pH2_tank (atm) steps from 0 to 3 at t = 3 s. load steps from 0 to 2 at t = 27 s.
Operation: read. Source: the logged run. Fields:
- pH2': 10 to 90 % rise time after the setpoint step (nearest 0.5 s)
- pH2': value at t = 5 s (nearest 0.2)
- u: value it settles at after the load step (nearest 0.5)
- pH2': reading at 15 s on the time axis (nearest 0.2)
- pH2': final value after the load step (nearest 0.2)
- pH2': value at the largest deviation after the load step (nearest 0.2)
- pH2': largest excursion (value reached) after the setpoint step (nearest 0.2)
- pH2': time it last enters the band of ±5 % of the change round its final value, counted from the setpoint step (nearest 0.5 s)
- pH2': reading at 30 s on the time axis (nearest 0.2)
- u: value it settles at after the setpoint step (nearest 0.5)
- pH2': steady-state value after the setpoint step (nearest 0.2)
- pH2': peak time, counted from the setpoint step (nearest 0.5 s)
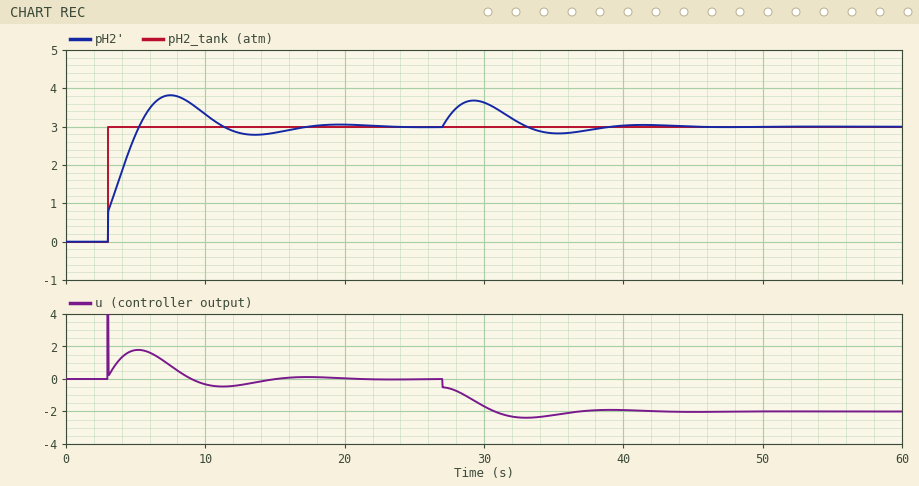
2.0 s
2.8
-2.0
2.8
3.0
3.6
3.8
12.0 s
3.6
0.0
3.0
4.5 s
